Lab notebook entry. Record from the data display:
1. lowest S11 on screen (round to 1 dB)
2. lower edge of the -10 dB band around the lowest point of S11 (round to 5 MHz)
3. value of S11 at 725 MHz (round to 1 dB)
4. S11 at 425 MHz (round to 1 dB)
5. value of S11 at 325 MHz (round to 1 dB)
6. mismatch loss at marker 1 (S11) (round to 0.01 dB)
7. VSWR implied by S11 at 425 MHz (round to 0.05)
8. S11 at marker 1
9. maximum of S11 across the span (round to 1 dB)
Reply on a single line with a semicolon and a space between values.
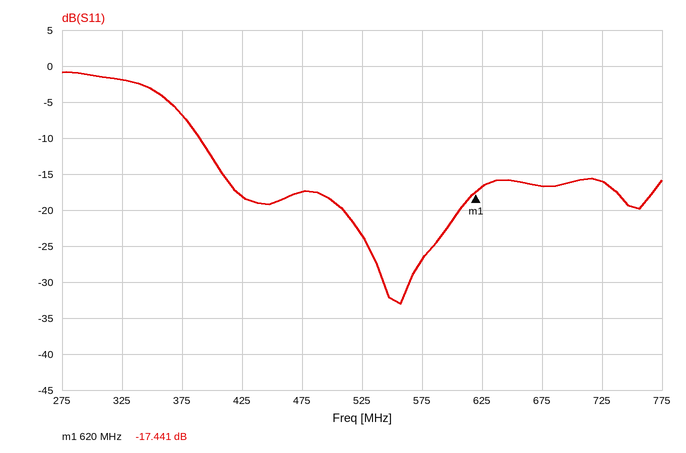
-33 dB; 390 MHz; -16 dB; -18 dB; -2 dB; 0.08 dB; 1.30; -17.441 dB; -1 dB
